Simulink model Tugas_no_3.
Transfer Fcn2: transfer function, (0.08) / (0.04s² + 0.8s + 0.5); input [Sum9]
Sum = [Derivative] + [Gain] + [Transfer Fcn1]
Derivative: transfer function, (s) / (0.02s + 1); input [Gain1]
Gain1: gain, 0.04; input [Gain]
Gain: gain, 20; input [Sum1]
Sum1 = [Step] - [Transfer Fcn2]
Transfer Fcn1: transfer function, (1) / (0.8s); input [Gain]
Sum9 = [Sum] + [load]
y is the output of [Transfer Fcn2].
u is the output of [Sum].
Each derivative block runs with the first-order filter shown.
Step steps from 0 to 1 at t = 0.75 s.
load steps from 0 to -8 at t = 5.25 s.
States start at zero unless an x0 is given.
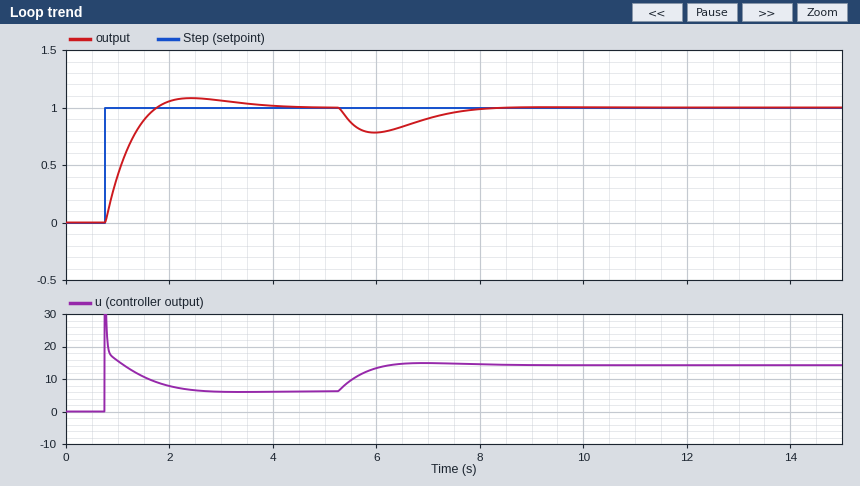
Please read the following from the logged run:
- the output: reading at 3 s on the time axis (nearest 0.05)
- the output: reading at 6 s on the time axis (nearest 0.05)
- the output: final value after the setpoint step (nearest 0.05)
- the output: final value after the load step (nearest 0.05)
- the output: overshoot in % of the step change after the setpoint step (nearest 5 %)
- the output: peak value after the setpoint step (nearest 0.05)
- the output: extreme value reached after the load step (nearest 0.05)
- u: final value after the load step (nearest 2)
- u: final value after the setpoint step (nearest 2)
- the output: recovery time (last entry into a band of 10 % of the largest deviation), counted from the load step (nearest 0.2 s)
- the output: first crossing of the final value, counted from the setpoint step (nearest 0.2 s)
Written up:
1.05
0.80
1.00
1.00
10 %
1.10
0.80
14
6
2.6 s
1.0 s
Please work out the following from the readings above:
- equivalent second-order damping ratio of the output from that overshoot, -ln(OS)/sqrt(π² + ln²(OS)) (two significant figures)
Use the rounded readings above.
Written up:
0.59
